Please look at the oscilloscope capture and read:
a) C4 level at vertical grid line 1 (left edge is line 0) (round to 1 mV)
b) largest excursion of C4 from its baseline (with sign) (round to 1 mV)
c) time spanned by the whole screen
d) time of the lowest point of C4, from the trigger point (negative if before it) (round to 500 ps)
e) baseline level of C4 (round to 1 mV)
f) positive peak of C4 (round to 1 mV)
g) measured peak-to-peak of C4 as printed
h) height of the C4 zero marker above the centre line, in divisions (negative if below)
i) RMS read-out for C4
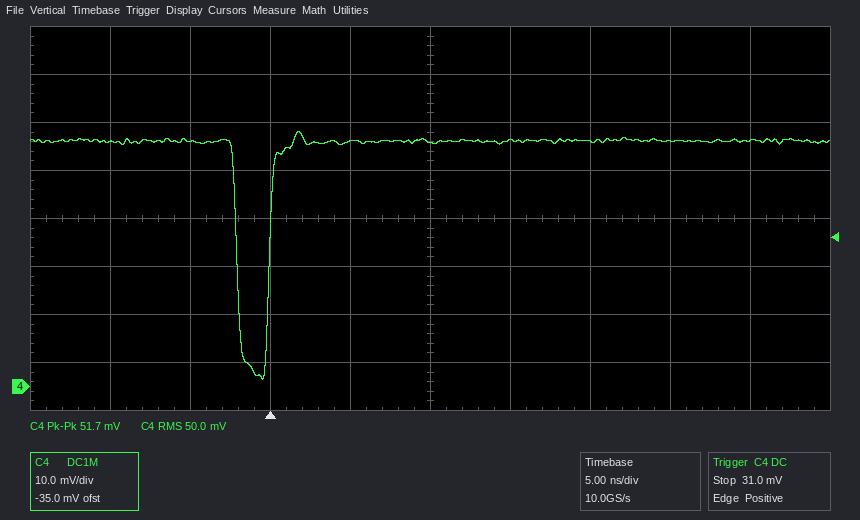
51 mV
-50 mV
50 ns
-500 ps
51 mV
53 mV
51.7 mV
-3.5 div
50.0 mV
